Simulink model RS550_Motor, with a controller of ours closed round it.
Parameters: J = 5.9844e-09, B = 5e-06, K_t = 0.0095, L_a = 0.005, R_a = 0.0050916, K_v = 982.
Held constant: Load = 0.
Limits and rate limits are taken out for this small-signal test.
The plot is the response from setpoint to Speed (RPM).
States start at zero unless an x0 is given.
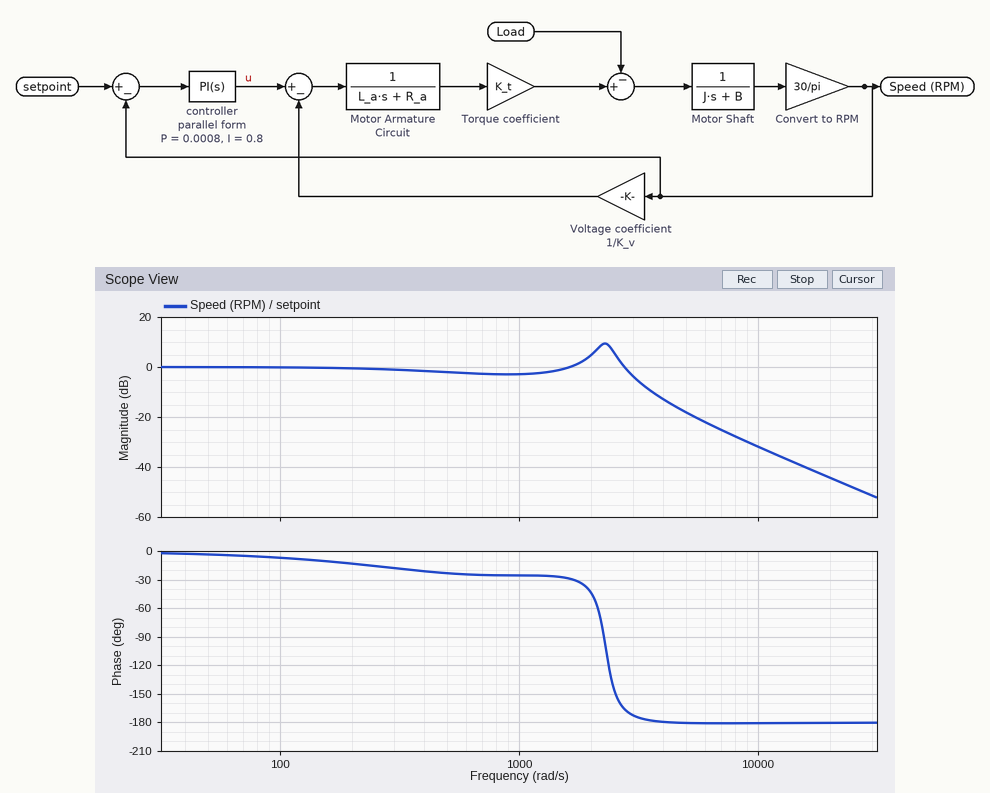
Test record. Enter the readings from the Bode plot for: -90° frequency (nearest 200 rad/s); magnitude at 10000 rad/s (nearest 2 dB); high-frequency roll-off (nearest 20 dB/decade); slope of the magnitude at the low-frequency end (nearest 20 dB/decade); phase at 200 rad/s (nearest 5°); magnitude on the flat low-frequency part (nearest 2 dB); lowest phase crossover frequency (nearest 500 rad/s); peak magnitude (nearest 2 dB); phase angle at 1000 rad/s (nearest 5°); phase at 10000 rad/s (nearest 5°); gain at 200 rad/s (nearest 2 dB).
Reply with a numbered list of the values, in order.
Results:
1. 2200 rad/s
2. -32 dB
3. -40 dB/decade
4. 0 dB/decade
5. -15°
6. 0 dB
7. 4500 rad/s
8. 10 dB
9. -25°
10. -180°
11. 0 dB
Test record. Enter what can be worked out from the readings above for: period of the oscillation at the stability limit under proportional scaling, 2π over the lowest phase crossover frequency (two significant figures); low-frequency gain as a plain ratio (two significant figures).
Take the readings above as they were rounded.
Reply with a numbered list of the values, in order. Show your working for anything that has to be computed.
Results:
1. 2π / 4500 = 0.0014 s
2. 10^(0 / 20) = 1.0
